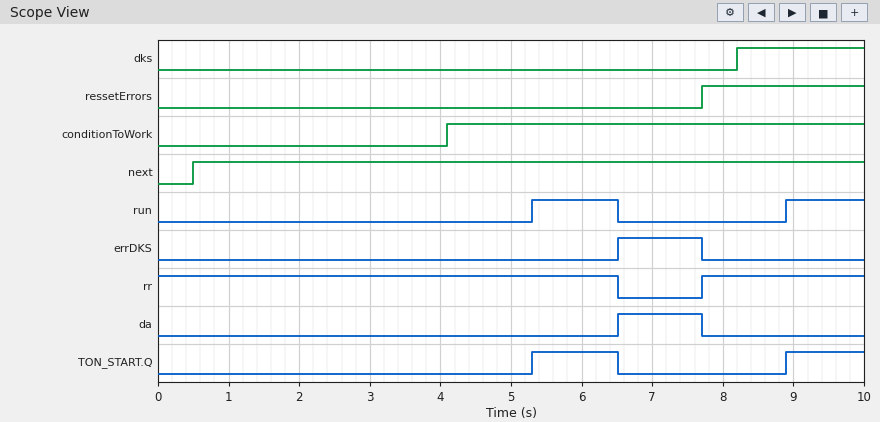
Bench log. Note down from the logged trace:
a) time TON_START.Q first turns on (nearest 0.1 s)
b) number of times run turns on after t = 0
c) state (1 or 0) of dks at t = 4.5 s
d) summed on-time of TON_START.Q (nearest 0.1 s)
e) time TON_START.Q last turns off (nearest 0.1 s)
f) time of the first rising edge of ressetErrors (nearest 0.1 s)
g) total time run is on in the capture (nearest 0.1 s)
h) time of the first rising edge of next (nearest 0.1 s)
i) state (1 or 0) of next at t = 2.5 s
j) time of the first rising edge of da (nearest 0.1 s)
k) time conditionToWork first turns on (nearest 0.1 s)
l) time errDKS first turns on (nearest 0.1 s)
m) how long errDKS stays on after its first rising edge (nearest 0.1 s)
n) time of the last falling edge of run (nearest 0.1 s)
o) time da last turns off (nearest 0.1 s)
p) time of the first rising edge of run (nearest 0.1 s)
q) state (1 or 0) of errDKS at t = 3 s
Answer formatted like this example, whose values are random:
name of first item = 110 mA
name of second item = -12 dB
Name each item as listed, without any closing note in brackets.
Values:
time TON_START.Q first turns on = 5.3 s
number of times run turns on after t = 0 = 2
state (1 or 0) of dks at t = 4.5 s = 0
summed on-time of TON_START.Q = 2.3 s
time TON_START.Q last turns off = 6.5 s
time of the first rising edge of ressetErrors = 7.7 s
total time run is on in the capture = 2.3 s
time of the first rising edge of next = 0.5 s
state (1 or 0) of next at t = 2.5 s = 1
time of the first rising edge of da = 6.5 s
time conditionToWork first turns on = 4.1 s
time errDKS first turns on = 6.5 s
how long errDKS stays on after its first rising edge = 1.2 s
time of the last falling edge of run = 6.5 s
time da last turns off = 7.7 s
time of the first rising edge of run = 5.3 s
state (1 or 0) of errDKS at t = 3 s = 0
